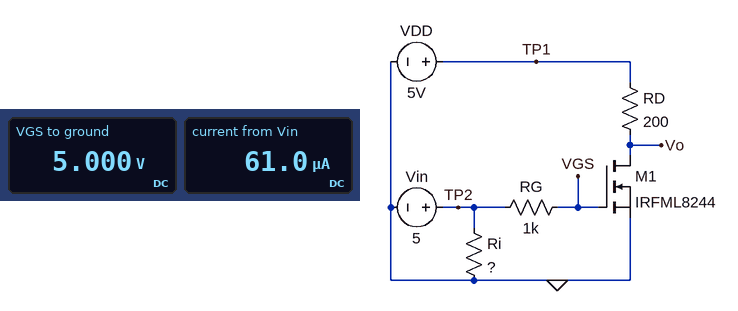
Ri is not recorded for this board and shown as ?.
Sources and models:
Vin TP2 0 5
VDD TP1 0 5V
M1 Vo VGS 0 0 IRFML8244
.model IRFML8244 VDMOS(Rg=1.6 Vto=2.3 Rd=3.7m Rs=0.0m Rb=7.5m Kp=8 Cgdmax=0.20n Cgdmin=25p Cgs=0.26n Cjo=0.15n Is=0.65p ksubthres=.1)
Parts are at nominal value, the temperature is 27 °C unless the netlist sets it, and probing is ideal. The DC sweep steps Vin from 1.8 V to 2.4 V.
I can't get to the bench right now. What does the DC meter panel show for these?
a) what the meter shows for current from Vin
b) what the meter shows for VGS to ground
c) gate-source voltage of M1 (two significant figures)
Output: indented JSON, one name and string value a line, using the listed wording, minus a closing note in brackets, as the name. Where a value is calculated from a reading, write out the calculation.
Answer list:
{
  "what the meter shows for current from Vin": "61.0 µA",
  "what the meter shows for VGS to ground": "5.000 V",
  "gate-source voltage of M1": "5 V = 5.0 V"
}
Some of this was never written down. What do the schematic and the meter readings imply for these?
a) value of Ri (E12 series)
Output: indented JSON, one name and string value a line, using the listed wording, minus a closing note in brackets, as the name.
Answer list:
{
  "value of Ri": "82 kΩ"
}
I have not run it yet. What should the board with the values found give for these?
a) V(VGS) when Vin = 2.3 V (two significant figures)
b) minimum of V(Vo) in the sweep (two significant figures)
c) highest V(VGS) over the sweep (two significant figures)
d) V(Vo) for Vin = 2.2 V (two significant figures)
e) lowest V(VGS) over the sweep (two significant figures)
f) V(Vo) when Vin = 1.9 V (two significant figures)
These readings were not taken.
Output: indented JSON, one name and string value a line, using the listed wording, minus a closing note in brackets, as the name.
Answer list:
{
  "V(VGS) when Vin = 2.3 V": "2.3 V",
  "minimum of V(Vo) in the sweep": "26 mV",
  "highest V(VGS) over the sweep": "2.4 V",
  "V(Vo) for Vin = 2.2 V": "4.2 V",
  "lowest V(VGS) over the sweep": "1.8 V",
  "V(Vo) when Vin = 1.9 V": "5.0 V"
}
